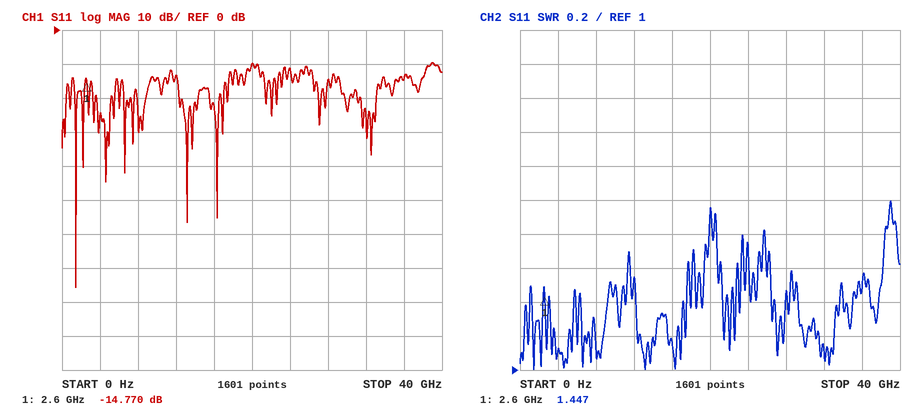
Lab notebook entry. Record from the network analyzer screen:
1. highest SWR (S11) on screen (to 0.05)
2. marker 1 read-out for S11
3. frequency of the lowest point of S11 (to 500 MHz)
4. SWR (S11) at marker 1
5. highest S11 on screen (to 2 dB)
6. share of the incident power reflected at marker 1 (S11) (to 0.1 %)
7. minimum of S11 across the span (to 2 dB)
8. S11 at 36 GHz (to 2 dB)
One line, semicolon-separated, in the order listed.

2.00; -14.770 dB; 1.5 GHz; 1.447; -10 dB; 3.3 %; -76 dB; -14 dB
